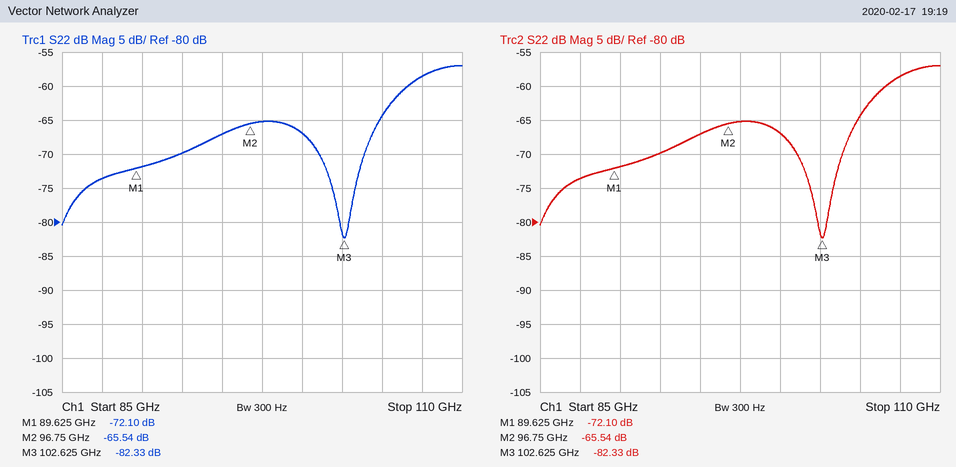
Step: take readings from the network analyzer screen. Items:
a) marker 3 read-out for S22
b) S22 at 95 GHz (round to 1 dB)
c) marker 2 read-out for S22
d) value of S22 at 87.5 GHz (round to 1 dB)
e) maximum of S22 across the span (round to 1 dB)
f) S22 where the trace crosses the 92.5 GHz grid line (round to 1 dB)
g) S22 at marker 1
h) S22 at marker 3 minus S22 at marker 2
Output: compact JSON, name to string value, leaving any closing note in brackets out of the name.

{"marker 3 read-out for S22": "-82.33 dB", "S22 at 95 GHz": "-67 dB", "marker 2 read-out for S22": "-65.54 dB", "value of S22 at 87.5 GHz": "-74 dB", "maximum of S22 across the span": "-57 dB", "S22 where the trace crosses the 92.5 GHz grid line": "-70 dB", "S22 at marker 1": "-72.10 dB", "S22 at marker 3 minus S22 at marker 2": "-16.79 dB"}
